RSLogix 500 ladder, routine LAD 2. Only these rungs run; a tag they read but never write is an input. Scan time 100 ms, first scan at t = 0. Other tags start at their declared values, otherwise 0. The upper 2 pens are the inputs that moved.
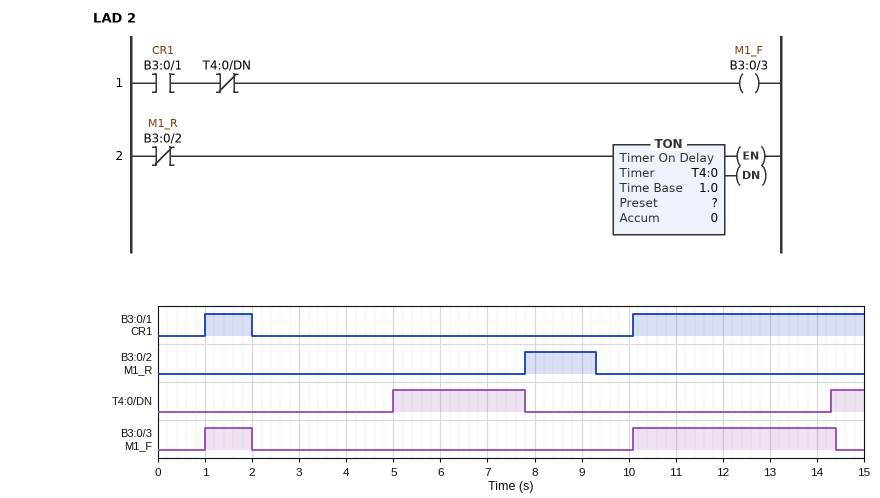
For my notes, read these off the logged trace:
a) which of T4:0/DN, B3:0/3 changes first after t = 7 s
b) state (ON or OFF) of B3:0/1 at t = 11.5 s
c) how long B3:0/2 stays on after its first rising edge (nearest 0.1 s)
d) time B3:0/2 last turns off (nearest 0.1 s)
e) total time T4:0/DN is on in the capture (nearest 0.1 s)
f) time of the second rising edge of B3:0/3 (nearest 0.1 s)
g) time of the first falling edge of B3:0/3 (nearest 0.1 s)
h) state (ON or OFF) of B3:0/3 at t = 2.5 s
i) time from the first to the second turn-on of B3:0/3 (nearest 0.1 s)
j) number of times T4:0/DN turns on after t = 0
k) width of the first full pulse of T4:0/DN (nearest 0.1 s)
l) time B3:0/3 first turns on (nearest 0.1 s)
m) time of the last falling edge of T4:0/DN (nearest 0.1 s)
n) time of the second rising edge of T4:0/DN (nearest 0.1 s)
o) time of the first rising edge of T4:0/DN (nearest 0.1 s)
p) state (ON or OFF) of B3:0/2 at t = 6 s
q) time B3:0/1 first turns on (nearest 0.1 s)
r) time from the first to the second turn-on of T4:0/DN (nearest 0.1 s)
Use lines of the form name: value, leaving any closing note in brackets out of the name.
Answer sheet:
which of T4:0/DN, B3:0/3 changes first after t = 7 s: T4:0/DN
state (ON or OFF) of B3:0/1 at t = 11.5 s: ON
how long B3:0/2 stays on after its first rising edge: 1.5 s
time B3:0/2 last turns off: 9.3 s
total time T4:0/DN is on in the capture: 3.5 s
time of the second rising edge of B3:0/3: 10.1 s
time of the first falling edge of B3:0/3: 2.0 s
state (ON or OFF) of B3:0/3 at t = 2.5 s: OFF
time from the first to the second turn-on of B3:0/3: 9.1 s
number of times T4:0/DN turns on after t = 0: 2
width of the first full pulse of T4:0/DN: 2.8 s
time B3:0/3 first turns on: 1.0 s
time of the last falling edge of T4:0/DN: 7.8 s
time of the second rising edge of T4:0/DN: 14.3 s
time of the first rising edge of T4:0/DN: 5.0 s
state (ON or OFF) of B3:0/2 at t = 6 s: OFF
time B3:0/1 first turns on: 1.0 s
time from the first to the second turn-on of T4:0/DN: 9.3 s
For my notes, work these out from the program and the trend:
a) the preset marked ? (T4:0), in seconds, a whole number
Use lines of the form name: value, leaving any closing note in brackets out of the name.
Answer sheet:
the preset marked ? (T4:0), in seconds, a whole number: 5 s
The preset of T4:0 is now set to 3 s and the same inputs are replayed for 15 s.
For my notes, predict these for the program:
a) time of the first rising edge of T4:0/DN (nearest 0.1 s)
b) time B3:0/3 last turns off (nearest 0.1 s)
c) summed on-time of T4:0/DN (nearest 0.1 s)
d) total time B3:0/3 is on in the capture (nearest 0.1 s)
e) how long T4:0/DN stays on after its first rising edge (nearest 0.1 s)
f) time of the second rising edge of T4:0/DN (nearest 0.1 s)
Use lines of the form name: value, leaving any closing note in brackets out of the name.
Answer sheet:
time of the first rising edge of T4:0/DN: 3.0 s
time B3:0/3 last turns off: 12.4 s
summed on-time of T4:0/DN: 7.5 s
total time B3:0/3 is on in the capture: 3.3 s
how long T4:0/DN stays on after its first rising edge: 4.8 s
time of the second rising edge of T4:0/DN: 12.3 s
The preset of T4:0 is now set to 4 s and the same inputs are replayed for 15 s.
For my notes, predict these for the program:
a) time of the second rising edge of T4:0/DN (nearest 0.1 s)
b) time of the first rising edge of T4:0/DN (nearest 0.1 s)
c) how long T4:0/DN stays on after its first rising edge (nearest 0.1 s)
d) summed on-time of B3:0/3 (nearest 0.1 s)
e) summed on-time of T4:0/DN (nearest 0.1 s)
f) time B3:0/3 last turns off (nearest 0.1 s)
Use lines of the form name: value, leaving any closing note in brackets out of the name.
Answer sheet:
time of the second rising edge of T4:0/DN: 13.3 s
time of the first rising edge of T4:0/DN: 4.0 s
how long T4:0/DN stays on after its first rising edge: 3.8 s
summed on-time of B3:0/3: 4.3 s
summed on-time of T4:0/DN: 5.5 s
time B3:0/3 last turns off: 13.4 s
